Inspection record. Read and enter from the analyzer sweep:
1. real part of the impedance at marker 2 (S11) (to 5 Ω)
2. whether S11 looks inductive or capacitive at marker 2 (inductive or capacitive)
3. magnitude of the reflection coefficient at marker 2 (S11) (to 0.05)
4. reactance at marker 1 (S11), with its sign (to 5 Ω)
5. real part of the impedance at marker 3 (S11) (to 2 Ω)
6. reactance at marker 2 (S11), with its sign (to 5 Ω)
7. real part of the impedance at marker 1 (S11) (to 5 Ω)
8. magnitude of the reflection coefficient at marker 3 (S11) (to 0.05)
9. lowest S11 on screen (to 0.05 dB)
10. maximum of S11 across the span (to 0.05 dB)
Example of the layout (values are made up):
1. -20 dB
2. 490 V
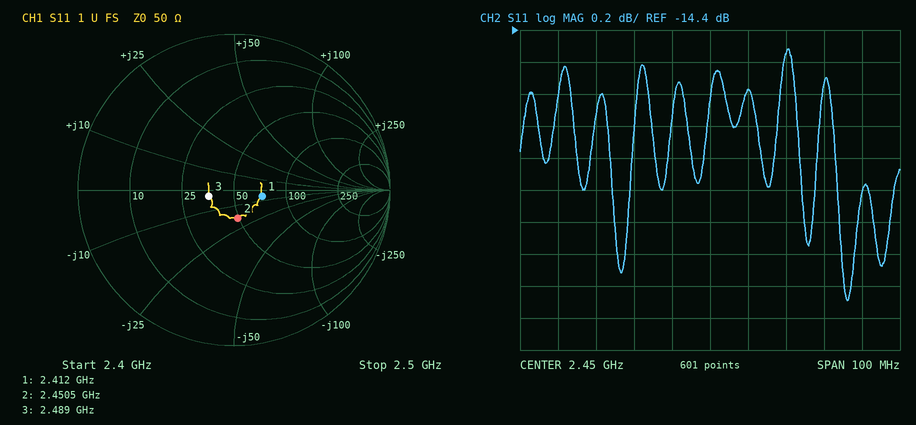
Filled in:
1. 50 Ω
2. capacitive
3. 0.20
4. -5 Ω
5. 36 Ω
6. -20 Ω
7. 70 Ω
8. 0.15
9. -16.10 dB
10. -14.50 dB
